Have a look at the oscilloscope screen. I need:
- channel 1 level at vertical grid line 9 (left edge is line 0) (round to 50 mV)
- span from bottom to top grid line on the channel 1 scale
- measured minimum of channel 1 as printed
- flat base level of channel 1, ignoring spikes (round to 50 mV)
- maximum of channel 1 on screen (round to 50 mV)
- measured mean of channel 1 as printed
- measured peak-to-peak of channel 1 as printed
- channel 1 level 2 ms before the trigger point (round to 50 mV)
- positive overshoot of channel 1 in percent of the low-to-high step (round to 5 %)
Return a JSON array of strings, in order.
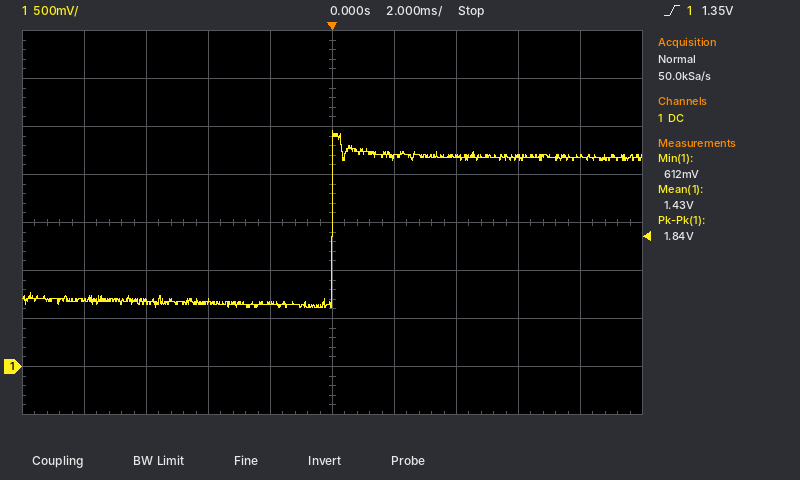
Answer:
["2.20 V", "4 V", "612 mV", "650 mV", "2.45 V", "1.43 V", "1.84 V", "650 mV", "20 %"]
